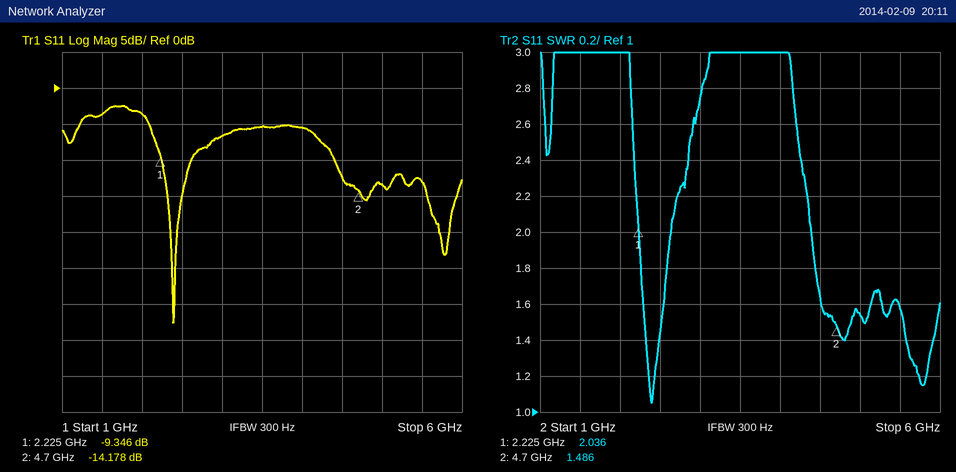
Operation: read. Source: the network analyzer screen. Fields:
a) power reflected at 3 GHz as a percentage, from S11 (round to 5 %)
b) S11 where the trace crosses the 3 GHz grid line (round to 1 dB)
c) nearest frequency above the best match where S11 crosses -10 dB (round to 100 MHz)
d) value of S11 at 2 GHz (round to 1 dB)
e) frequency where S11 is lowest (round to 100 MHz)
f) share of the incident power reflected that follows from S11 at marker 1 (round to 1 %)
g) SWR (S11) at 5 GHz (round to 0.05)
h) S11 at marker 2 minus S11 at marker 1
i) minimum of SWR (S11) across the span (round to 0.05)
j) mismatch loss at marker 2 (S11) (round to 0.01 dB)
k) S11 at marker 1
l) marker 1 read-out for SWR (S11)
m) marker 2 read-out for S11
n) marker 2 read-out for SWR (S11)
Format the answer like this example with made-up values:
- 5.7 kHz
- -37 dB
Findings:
- 20 %
- -7 dB
- 2.6 GHz
- -4 dB
- 2.4 GHz
- 12 %
- 1.55
- -4.832 dB
- 1.05
- 0.17 dB
- -9.346 dB
- 2.036
- -14.178 dB
- 1.486
